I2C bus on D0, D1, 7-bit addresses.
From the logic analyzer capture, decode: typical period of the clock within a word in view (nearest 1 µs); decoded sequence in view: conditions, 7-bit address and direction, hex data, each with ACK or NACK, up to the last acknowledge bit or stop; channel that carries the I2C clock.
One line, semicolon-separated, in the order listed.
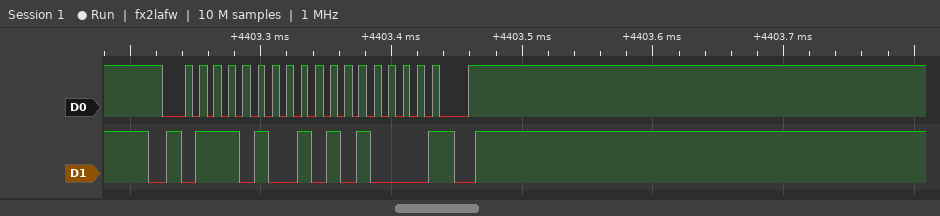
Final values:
11 µs; start, address 3A write NACK, 50 NACK, stop; D0
